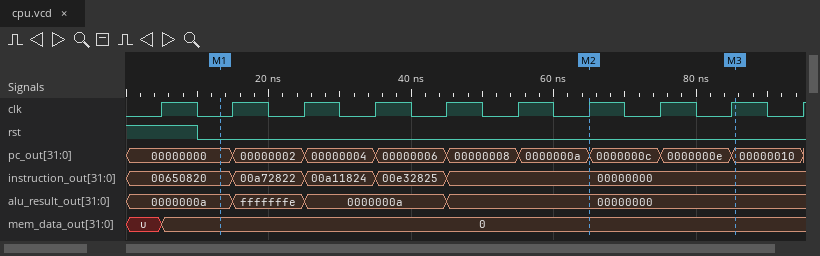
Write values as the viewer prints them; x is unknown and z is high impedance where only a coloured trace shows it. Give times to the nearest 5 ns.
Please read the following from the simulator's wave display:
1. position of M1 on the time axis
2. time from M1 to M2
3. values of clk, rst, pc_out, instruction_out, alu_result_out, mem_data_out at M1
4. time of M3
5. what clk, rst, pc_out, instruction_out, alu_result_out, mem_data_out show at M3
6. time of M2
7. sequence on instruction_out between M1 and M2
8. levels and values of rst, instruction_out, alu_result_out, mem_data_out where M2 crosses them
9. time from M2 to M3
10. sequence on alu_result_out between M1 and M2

15 ns
50 ns
clk=0, rst=0, pc_out=00000000, instruction_out=00650820, alu_result_out=0000000a, mem_data_out=0
85 ns
clk=1, rst=0, pc_out=00000010, instruction_out=00000000, alu_result_out=00000000, mem_data_out=0
65 ns
00650820, 00a72822, 00a11824, 00e32825, 00000000
rst=0, instruction_out=00000000, alu_result_out=00000000, mem_data_out=0
20 ns
0000000a, fffffffe, 0000000a, 00000000
